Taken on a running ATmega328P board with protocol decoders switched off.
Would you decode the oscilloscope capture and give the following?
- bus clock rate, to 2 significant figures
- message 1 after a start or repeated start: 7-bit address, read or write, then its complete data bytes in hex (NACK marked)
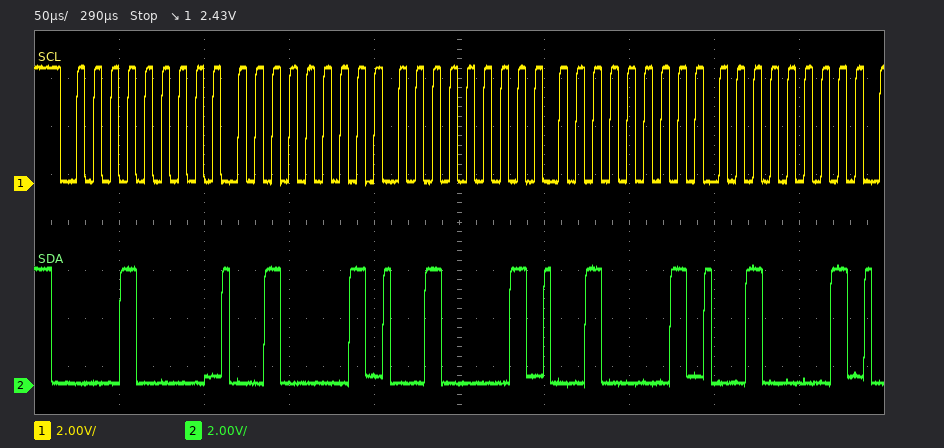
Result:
100 kHz
0x08 write: 21 21 21 21
